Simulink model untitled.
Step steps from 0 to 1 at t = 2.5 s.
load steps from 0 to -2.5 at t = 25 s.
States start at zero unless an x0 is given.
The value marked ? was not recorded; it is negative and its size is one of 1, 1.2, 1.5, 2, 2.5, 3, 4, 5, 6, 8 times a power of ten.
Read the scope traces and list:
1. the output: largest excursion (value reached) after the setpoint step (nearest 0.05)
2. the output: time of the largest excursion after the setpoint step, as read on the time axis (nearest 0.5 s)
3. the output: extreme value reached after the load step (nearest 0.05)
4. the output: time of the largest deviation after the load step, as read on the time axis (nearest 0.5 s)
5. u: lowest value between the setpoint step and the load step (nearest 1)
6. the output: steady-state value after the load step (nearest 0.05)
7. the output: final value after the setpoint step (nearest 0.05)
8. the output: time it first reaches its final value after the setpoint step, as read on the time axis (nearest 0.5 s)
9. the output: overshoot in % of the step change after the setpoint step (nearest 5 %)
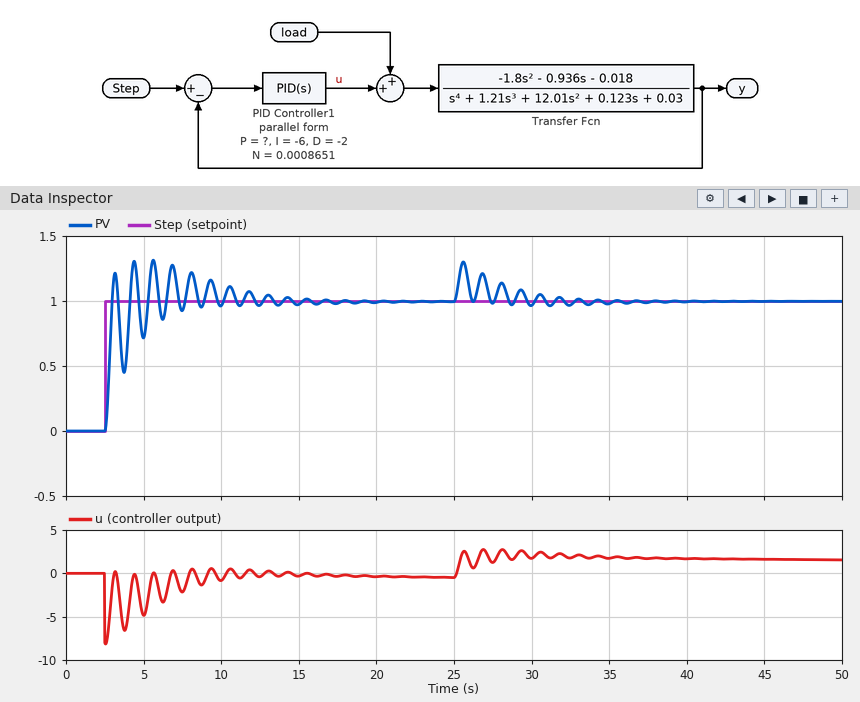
1.30
5.5 s
1.30
25.5 s
-8
1.00
1.00
3.0 s
30 %
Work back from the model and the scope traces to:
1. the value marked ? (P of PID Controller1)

-8
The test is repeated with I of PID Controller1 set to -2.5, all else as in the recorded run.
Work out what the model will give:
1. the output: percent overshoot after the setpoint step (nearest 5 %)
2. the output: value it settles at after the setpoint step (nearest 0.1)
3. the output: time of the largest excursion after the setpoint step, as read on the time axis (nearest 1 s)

15 %
1.0
7 s
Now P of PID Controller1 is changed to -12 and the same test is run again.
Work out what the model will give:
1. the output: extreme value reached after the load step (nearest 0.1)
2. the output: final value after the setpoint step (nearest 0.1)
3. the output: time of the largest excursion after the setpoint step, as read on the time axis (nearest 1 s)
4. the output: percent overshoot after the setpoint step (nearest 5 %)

1.2
1.0
4 s
35 %
